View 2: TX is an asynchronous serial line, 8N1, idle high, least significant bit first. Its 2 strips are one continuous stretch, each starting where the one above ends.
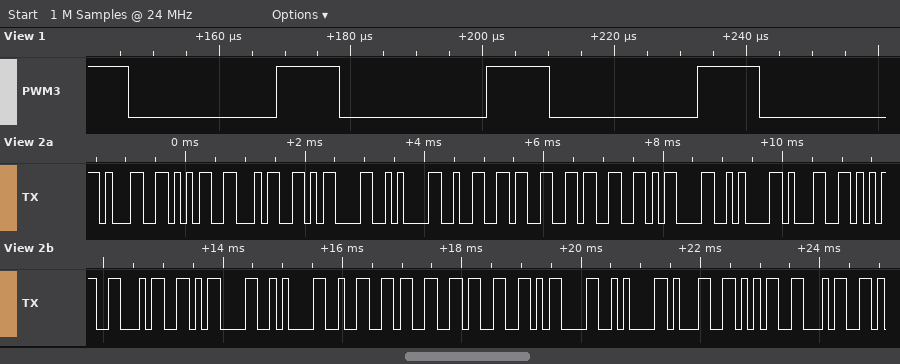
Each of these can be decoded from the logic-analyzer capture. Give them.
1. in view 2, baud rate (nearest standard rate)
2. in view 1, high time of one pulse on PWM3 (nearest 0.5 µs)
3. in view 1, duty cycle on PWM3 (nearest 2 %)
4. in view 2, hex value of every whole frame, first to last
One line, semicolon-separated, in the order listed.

9600 baud; 9.5 µs; 30 %; 31 35 34 0D 0A 32 33 33 0D 0A 31 35 34 0D 0A 32 33 33 0D 0A 31 35 34
